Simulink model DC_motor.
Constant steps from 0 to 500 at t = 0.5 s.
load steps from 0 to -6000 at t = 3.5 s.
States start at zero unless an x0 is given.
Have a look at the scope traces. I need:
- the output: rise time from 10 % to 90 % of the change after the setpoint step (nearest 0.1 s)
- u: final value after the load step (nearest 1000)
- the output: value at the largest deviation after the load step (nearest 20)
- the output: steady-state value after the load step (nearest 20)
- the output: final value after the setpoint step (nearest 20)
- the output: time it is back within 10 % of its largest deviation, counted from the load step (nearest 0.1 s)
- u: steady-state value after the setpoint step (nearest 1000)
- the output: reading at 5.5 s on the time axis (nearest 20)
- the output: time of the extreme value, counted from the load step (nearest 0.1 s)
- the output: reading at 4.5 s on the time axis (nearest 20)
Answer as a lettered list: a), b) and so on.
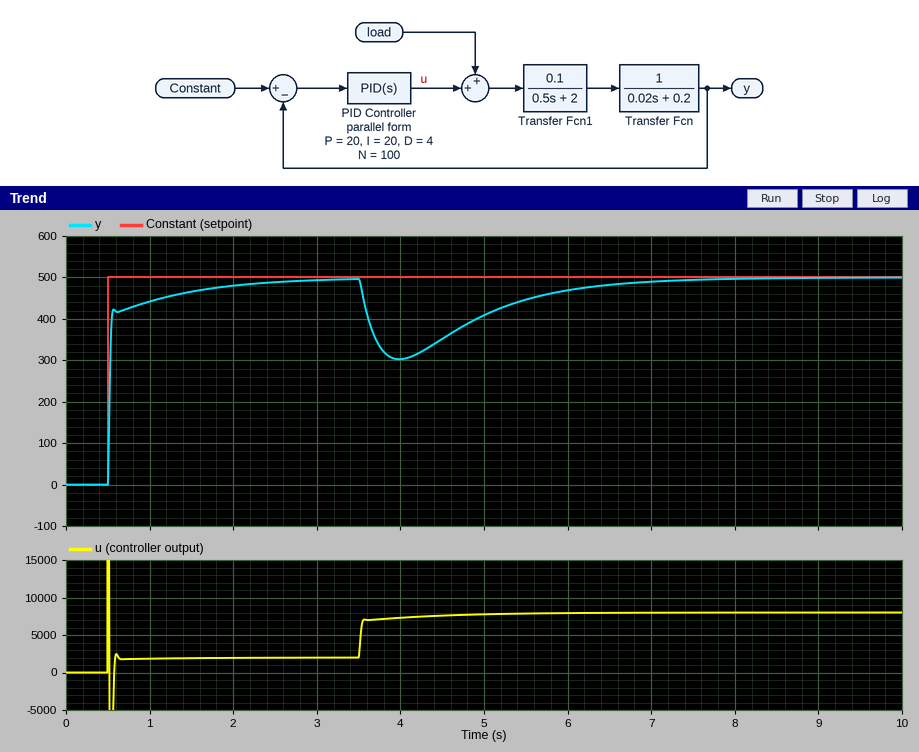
a) 0.6 s
b) 8000
c) 300
d) 500
e) 500
f) 2.9 s
g) 2000
h) 440
i) 0.5 s
j) 360
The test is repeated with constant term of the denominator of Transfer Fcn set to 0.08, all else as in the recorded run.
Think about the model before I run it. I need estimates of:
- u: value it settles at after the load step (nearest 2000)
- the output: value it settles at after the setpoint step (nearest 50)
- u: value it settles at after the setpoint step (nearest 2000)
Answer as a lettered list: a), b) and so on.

a) 6000
b) 500
c) 0
